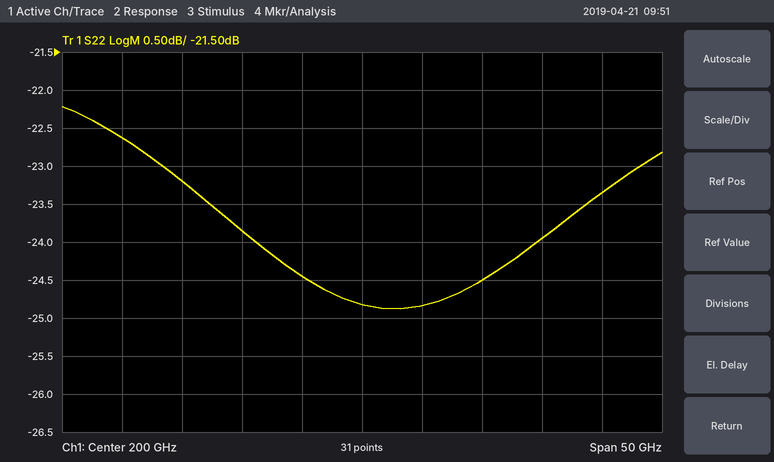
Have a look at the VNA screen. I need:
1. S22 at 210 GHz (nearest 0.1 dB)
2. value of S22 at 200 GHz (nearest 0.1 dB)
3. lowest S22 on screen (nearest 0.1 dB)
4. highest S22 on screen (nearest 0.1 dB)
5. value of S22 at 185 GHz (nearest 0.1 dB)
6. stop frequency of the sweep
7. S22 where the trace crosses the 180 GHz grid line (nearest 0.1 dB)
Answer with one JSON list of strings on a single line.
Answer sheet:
["-24.5 dB", "-24.8 dB", "-24.9 dB", "-22.2 dB", "-23.2 dB", "225 GHz", "-22.6 dB"]
